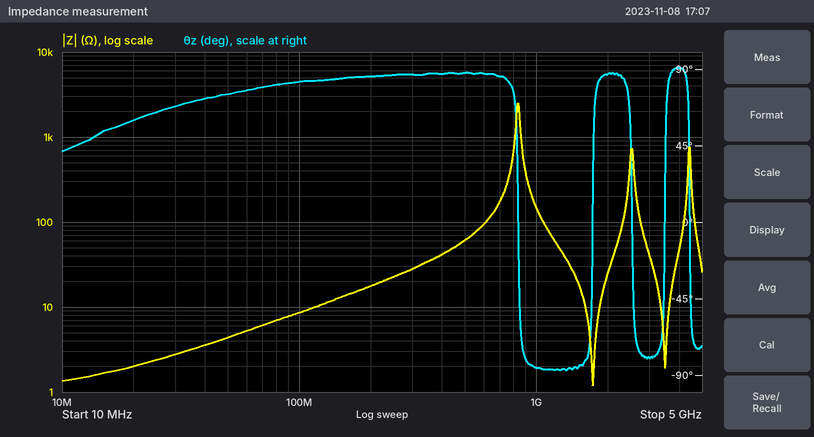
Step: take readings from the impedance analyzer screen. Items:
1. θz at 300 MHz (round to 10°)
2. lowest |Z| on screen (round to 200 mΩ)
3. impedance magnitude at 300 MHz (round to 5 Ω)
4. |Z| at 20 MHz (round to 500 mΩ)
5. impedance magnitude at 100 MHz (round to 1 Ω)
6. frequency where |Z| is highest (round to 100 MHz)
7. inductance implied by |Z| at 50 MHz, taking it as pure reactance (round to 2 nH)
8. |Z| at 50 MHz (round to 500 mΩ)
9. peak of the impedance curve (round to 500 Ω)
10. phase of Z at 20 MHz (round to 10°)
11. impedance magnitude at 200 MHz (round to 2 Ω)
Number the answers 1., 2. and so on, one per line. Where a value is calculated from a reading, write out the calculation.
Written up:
1. 90°
2. 1.2 Ω
3. 30 Ω
4. 2.0 Ω
5. 9 Ω
6. 800 MHz
7. L = 4.5 Ω/(2π × 50 MHz) ≈ 14 nH
8. 4.5 Ω
9. 2.5 kΩ
10. 60°
11. 18 Ω
